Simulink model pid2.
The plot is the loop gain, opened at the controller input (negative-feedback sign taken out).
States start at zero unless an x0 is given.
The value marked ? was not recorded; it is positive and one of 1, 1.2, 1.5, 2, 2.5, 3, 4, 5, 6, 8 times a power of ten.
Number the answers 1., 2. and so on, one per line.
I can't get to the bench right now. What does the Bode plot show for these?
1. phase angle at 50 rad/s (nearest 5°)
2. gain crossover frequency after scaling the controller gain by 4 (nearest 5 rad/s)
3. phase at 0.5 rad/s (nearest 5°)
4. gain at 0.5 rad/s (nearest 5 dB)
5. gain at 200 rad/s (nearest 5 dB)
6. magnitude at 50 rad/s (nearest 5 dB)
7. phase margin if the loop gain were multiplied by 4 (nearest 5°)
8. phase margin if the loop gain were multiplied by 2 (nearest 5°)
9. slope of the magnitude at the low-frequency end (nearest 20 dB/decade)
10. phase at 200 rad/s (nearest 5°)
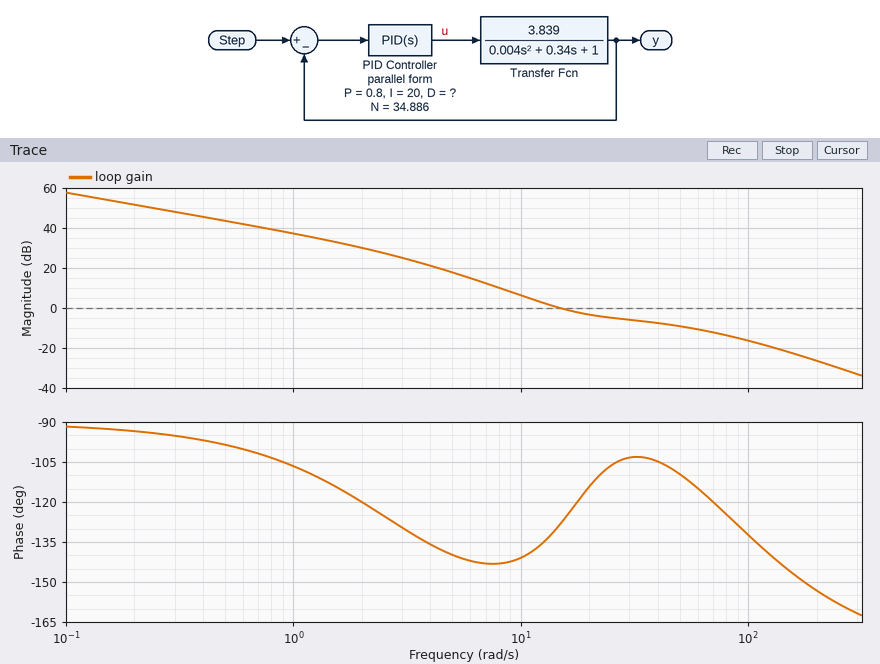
1. -110°
2. 70 rad/s
3. -100°
4. 45 dB
5. -25 dB
6. -10 dB
7. 60°
8. 75°
9. -20 dB/decade
10. -155°
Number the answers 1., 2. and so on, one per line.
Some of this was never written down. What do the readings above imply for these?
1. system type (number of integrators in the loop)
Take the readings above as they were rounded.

1. 1
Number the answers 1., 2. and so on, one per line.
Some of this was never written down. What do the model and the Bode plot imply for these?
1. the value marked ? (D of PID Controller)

1. 0.04
